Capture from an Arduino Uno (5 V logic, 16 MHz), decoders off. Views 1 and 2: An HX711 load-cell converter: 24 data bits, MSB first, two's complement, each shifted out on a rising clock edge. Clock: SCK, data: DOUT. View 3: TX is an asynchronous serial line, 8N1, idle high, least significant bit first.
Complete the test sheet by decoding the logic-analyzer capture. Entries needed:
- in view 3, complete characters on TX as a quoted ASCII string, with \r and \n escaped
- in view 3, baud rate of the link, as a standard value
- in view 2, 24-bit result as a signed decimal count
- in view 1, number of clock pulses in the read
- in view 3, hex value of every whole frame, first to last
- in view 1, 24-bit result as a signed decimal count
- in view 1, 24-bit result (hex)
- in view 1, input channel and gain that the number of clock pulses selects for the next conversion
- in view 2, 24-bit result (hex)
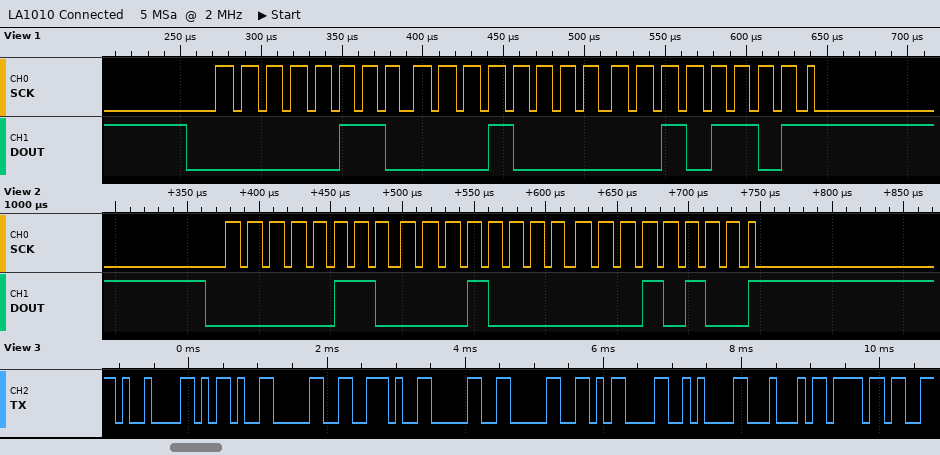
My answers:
"\t-0.00\r\nDo"
9600 baud
397332
25
09 2D 30 2E 30 30 0D 0A 44 6F
397357
0x06102D
channel A, gain 128
0x061014
